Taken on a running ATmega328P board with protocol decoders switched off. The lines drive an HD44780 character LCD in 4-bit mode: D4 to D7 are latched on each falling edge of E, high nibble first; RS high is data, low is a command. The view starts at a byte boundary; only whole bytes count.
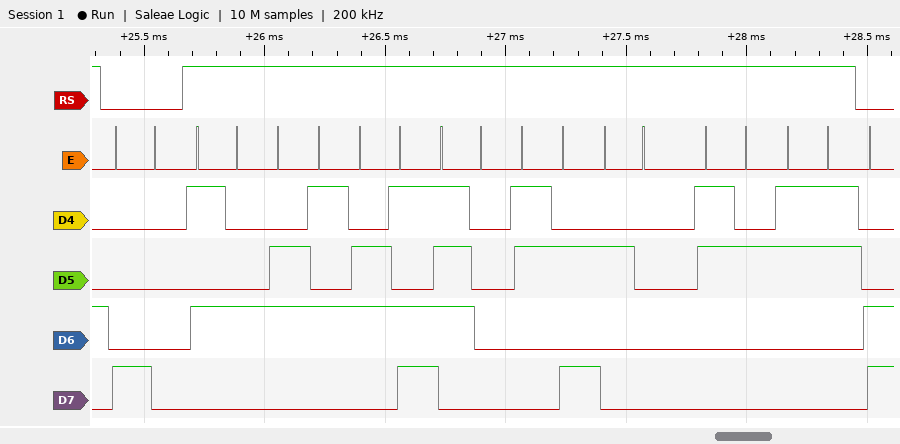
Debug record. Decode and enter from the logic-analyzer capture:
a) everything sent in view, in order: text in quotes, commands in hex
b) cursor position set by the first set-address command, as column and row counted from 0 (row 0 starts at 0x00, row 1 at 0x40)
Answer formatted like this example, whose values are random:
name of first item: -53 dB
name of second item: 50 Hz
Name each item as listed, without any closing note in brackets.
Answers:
everything sent in view, in order: text in quotes, commands in hex: 0x80 "Temp: 23"
cursor position set by the first set-address command, as column and row counted from 0: column 0, row 0
